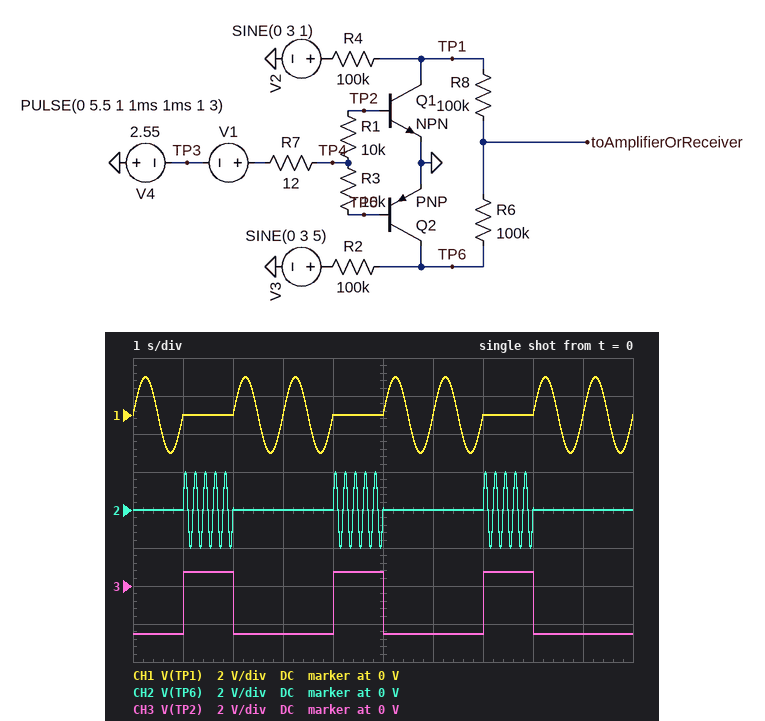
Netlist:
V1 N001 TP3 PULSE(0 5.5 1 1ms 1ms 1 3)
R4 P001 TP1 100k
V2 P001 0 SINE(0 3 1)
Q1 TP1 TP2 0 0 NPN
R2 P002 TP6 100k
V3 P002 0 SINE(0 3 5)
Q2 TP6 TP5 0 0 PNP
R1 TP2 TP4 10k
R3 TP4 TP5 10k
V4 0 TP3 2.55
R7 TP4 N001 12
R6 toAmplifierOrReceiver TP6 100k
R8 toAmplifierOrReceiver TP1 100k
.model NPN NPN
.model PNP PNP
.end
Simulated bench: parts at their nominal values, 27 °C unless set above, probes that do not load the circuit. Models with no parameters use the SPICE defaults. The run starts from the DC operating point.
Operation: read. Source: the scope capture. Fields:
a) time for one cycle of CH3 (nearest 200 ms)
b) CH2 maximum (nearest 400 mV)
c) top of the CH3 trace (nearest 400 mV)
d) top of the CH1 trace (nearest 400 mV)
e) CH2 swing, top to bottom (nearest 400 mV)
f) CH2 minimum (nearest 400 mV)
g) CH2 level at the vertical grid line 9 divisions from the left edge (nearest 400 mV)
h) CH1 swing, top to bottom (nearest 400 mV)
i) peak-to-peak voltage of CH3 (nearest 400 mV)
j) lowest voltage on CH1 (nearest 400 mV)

3.0 s
2.0 V
800 mV
2.0 V
4.0 V
-2.0 V
0 V
4.0 V
3.2 V
-2.0 V
